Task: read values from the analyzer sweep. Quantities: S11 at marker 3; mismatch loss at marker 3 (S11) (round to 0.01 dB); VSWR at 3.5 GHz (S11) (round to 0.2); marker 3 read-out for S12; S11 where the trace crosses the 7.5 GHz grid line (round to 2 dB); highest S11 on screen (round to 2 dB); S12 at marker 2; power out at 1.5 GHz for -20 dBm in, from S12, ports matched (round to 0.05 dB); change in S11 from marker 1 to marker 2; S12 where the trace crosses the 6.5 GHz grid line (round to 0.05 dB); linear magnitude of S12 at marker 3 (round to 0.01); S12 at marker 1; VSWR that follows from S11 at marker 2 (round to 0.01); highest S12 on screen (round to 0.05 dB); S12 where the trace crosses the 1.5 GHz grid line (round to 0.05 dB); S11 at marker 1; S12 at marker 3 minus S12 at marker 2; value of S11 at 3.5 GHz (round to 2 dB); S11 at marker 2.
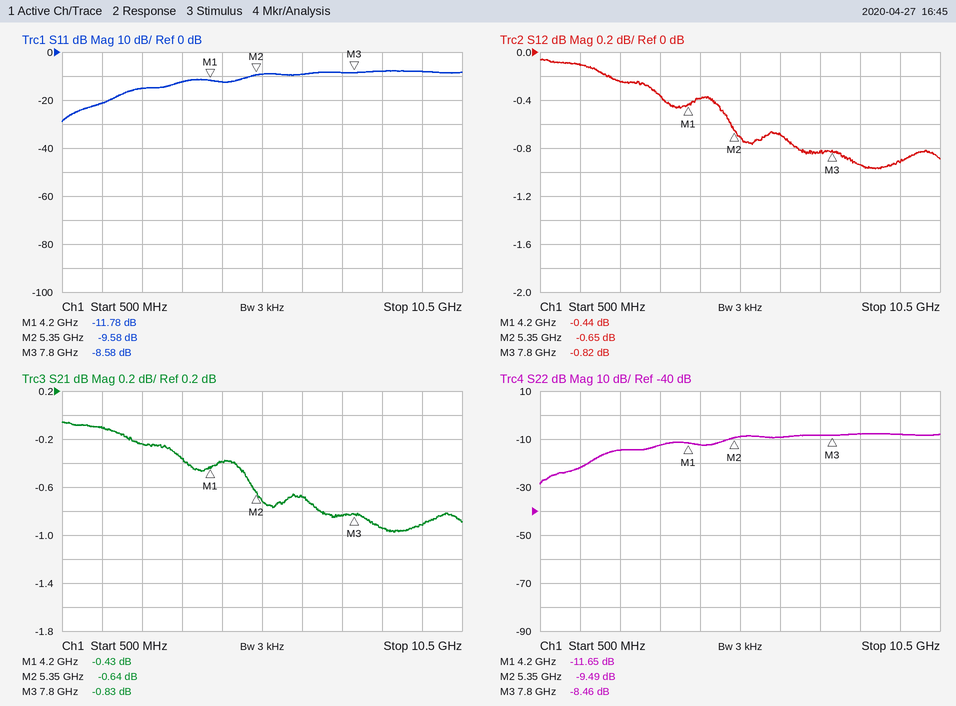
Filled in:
-8.58 dB
0.65 dB
1.6
-0.82 dB
-8 dB
-8 dB
-0.65 dB
-20.10 dBm
2.20 dB
-0.70 dB
0.91
-0.44 dB
1.99
-0.05 dB
-0.10 dB
-11.78 dB
-0.17 dB
-12 dB
-9.58 dB
